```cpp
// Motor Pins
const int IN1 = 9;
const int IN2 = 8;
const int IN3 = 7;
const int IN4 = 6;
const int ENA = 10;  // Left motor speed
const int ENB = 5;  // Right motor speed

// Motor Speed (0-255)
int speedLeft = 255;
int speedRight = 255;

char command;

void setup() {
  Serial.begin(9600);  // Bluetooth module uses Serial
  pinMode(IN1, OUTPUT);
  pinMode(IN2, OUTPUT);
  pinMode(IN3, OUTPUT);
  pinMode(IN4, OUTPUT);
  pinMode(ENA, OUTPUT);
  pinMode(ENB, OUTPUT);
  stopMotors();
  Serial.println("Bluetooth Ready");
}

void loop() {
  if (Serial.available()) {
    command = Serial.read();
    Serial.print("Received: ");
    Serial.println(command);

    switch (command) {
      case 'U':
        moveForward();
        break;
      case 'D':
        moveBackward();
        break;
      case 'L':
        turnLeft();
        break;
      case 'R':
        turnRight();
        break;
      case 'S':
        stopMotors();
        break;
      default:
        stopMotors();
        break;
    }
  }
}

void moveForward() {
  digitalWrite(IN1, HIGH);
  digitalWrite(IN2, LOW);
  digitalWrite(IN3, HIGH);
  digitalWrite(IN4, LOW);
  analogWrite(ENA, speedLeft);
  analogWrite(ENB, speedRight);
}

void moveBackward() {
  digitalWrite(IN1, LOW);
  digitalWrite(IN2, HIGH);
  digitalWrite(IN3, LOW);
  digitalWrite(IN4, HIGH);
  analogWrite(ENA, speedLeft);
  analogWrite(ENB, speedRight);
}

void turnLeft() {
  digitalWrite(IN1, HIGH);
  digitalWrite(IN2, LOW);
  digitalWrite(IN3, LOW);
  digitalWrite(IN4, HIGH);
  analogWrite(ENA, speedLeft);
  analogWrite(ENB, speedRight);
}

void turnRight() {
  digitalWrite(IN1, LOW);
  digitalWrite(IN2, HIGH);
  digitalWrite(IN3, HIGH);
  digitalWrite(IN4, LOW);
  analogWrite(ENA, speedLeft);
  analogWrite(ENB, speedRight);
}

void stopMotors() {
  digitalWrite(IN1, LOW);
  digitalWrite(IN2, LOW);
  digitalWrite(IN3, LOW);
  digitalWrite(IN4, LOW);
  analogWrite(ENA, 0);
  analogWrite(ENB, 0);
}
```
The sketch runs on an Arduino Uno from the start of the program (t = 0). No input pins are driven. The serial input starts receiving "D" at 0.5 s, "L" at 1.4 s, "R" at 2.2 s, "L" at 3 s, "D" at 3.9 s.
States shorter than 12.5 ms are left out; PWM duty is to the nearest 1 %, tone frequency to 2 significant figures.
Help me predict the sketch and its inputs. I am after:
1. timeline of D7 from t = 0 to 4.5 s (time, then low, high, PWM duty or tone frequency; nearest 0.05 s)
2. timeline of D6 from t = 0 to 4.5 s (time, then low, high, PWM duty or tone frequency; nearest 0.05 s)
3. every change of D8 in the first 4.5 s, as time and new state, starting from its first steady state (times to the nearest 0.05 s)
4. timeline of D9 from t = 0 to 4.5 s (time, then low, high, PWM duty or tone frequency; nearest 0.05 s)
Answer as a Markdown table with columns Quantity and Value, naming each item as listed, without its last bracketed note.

| Quantity | Value |
|---|---|
| timeline of D7 from t = 0 to 4.5 s | 0 s low; 2.2 s high; 3 s low |
| timeline of D6 from t = 0 to 4.5 s | 0 s low; 0.5 s high; 2.2 s low; 3 s high |
| every change of D8 in the first 4.5 s, as time and new state, starting from its first steady state | 0 s low; 0.5 s high; 1.4 s low; 2.2 s high; 3 s low; 3.9 s high |
| timeline of D9 from t = 0 to 4.5 s | 0 s low; 1.4 s high; 2.2 s low; 3 s high; 3.9 s low |
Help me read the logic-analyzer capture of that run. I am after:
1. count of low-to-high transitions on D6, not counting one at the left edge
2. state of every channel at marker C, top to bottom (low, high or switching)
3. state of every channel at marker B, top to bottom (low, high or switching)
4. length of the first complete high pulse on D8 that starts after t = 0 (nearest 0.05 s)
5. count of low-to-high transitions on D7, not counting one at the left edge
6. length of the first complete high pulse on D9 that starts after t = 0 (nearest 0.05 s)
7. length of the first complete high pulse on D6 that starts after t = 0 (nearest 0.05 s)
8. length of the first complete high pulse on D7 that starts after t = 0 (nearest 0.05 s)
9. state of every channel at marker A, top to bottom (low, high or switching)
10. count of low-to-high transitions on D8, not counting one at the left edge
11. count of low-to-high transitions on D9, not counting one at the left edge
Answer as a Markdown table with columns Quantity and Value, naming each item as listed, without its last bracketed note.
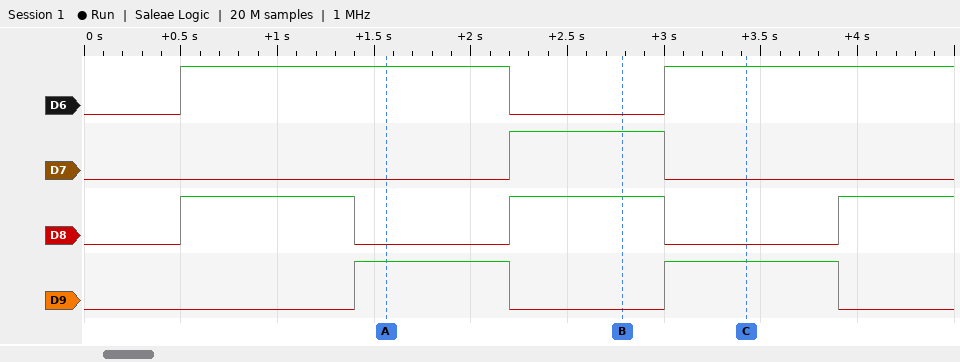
| Quantity | Value |
|---|---|
| count of low-to-high transitions on D6, not counting one at the left edge | 2 |
| state of every channel at marker C, top to bottom | D6 high, D7 low, D8 low, D9 high |
| state of every channel at marker B, top to bottom | D6 low, D7 high, D8 high, D9 low |
| length of the first complete high pulse on D8 that starts after t = 0 | 0.90 s |
| count of low-to-high transitions on D7, not counting one at the left edge | 1 |
| length of the first complete high pulse on D9 that starts after t = 0 | 0.80 s |
| length of the first complete high pulse on D6 that starts after t = 0 | 1.70 s |
| length of the first complete high pulse on D7 that starts after t = 0 | 0.80 s |
| state of every channel at marker A, top to bottom | D6 high, D7 low, D8 low, D9 high |
| count of low-to-high transitions on D8, not counting one at the left edge | 3 |
| count of low-to-high transitions on D9, not counting one at the left edge | 2 |
